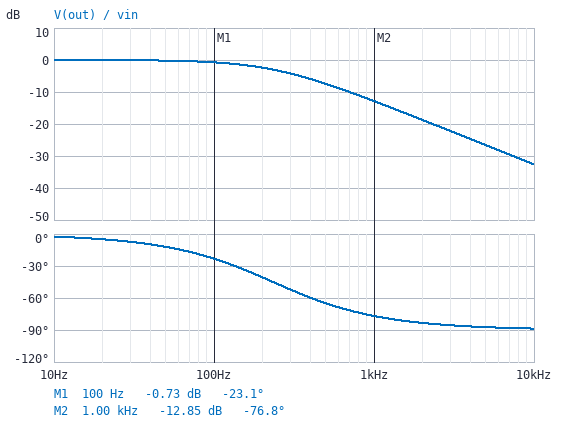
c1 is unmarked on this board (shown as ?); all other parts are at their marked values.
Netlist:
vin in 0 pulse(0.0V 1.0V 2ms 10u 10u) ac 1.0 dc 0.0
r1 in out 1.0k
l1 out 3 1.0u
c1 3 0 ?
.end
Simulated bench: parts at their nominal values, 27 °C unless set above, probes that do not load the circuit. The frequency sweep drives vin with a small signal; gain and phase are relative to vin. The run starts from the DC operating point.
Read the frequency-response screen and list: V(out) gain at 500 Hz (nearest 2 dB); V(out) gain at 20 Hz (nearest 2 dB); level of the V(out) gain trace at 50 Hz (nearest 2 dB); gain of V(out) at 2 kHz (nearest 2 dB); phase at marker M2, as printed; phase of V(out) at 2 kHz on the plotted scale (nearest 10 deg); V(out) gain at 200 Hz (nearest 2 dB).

-8 dB
0 dB
0 dB
-18 dB
-76.8 deg
-80 deg
-2 dB
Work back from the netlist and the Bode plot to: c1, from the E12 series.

680 nF
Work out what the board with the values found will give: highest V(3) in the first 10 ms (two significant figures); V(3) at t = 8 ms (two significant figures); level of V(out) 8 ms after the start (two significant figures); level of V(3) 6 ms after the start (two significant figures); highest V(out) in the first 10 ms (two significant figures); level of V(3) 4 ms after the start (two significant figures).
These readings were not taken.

1.0 V
1.0 V
1.0 V
1.0 V
1.0 V
950 mV
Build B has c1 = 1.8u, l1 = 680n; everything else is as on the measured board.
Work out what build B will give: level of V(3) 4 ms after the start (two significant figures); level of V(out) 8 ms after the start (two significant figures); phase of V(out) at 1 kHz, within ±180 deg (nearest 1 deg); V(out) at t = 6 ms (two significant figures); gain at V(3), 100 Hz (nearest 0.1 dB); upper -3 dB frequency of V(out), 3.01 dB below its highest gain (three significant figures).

670 mV
960 mV
-85 deg
890 mV
-3.6 dB
88.4 Hz
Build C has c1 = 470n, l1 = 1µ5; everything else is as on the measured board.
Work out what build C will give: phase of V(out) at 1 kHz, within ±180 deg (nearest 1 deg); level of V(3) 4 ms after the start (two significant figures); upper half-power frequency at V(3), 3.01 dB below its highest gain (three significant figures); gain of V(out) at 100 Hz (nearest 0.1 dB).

-71 deg
990 mV
339 Hz
-0.4 dB
